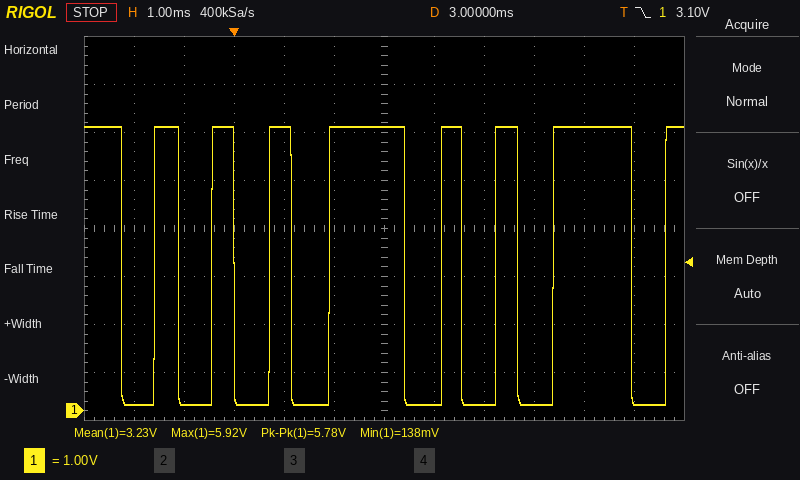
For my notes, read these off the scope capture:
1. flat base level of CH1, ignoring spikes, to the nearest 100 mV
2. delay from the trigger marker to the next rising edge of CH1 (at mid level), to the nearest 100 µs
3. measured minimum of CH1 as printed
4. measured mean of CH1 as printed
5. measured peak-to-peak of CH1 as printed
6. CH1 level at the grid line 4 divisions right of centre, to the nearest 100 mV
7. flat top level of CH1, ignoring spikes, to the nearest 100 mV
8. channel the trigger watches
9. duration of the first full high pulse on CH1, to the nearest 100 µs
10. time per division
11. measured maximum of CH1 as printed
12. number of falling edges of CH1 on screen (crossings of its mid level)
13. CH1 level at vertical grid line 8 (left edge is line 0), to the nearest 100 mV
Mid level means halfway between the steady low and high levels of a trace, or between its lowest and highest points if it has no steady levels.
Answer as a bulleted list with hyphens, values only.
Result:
- 100 mV
- 700 µs
- 138 mV
- 3.23 V
- 5.78 V
- 5.9 V
- 5.9 V
- CH1
- 500 µs
- 1 ms
- 5.92 V
- 8
- 100 mV
